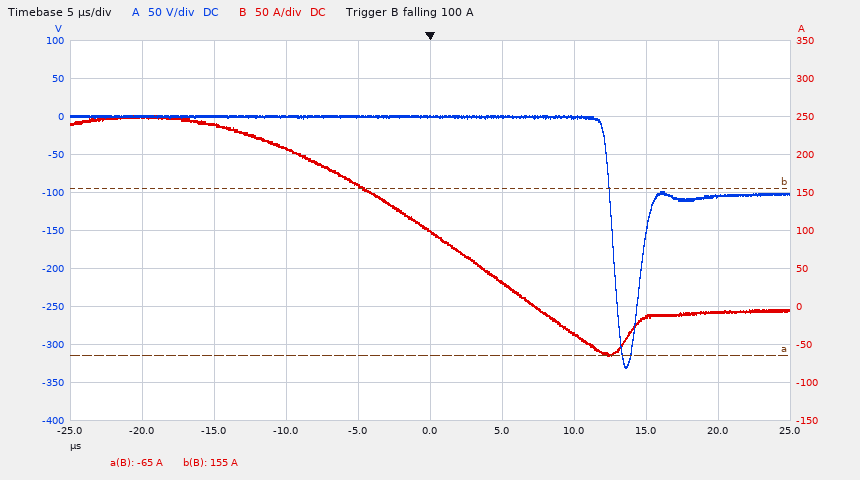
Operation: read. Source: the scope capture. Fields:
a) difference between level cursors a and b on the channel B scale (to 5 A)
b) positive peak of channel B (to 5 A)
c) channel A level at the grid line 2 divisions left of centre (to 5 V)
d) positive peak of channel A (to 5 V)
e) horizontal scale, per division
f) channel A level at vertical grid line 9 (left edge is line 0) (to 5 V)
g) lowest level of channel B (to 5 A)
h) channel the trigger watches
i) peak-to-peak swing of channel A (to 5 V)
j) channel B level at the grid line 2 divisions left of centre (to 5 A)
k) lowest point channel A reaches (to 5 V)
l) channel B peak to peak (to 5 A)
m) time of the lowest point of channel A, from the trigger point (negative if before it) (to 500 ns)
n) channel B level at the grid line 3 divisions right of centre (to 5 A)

220 A
250 A
0 V
0 V
5 µs
-105 V
-65 A
channel B
330 V
210 A
-330 V
315 A
+13.5 µs
-15 A
